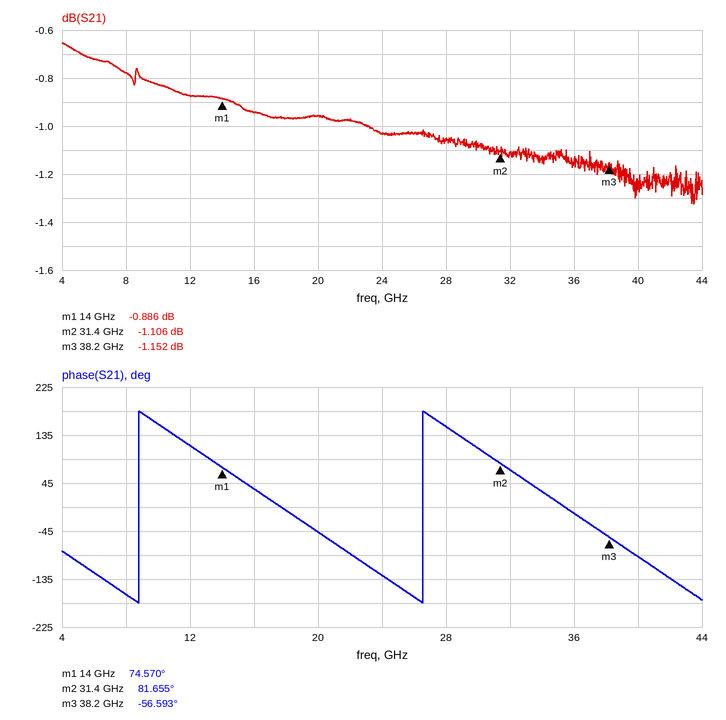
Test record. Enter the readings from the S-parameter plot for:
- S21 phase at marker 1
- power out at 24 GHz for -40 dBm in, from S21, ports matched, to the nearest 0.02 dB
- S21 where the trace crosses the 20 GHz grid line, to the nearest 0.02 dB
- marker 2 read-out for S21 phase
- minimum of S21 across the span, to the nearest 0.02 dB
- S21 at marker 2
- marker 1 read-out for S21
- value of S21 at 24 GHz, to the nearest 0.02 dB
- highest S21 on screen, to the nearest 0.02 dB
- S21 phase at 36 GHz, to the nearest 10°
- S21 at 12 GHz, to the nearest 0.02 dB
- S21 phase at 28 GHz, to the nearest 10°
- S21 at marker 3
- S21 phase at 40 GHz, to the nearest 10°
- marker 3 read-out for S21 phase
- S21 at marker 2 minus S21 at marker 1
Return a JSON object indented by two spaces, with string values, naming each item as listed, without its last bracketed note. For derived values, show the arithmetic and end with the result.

{
  "S21 phase at marker 1": "74.570°",
  "power out at 24 GHz for -40 dBm in, from S21, ports matched, to the nearest 0.02 dB": "-40 dBm + (-1.04 dB) = -41.04 dBm",
  "S21 where the trace crosses the 20 GHz grid line, to the nearest 0.02 dB": "-0.96 dB",
  "marker 2 read-out for S21 phase": "81.655°",
  "minimum of S21 across the span, to the nearest 0.02 dB": "-1.32 dB",
  "S21 at marker 2": "-1.106 dB",
  "marker 1 read-out for S21": "-0.886 dB",
  "value of S21 at 24 GHz, to the nearest 0.02 dB": "-1.04 dB",
  "highest S21 on screen, to the nearest 0.02 dB": "-0.66 dB",
  "S21 phase at 36 GHz, to the nearest 10°": "-10°",
  "S21 at 12 GHz, to the nearest 0.02 dB": "-0.88 dB",
  "S21 phase at 28 GHz, to the nearest 10°": "150°",
  "S21 at marker 3": "-1.152 dB",
  "S21 phase at 40 GHz, to the nearest 10°": "-90°",
  "marker 3 read-out for S21 phase": "-56.593°",
  "S21 at marker 2 minus S21 at marker 1": "-1.106 − (-0.886) = -0.220 dB"
}
